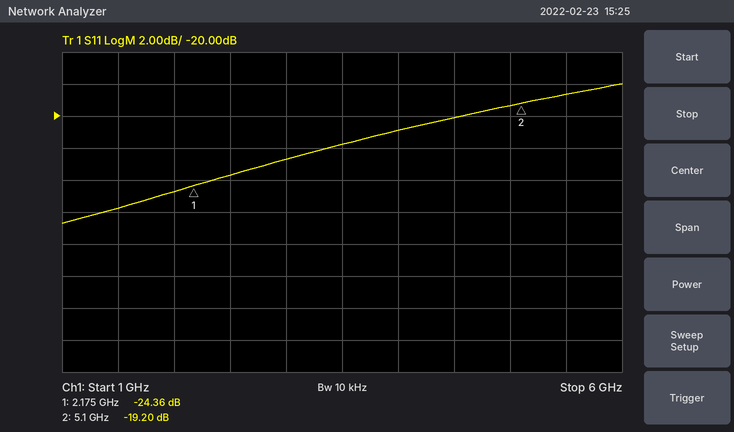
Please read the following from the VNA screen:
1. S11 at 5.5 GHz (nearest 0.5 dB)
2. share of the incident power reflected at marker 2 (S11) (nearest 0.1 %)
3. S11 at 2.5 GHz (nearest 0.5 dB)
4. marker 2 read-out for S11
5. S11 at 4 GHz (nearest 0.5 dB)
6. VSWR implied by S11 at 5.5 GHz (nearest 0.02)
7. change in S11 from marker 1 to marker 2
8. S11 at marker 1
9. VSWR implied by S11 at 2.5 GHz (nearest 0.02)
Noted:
-18.5 dB
1.2 %
-23.5 dB
-19.20 dB
-21.0 dB
1.26
5.16 dB
-24.36 dB
1.14
